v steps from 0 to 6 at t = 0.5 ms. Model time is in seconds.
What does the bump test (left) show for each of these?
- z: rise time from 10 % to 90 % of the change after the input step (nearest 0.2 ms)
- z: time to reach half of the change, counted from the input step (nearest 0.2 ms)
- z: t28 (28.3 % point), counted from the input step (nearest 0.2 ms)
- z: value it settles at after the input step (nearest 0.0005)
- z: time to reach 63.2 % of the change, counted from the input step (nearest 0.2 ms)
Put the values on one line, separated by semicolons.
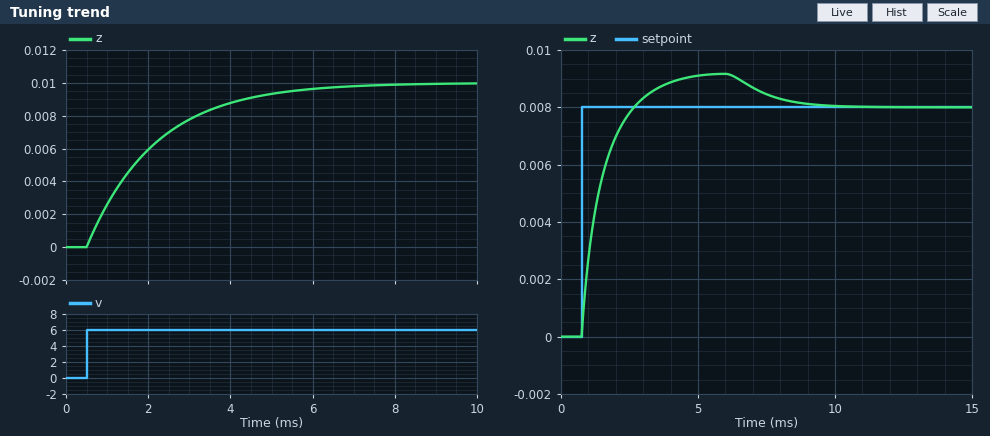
3.6 ms; 1.2 ms; 0.6 ms; 0.0100; 1.6 ms
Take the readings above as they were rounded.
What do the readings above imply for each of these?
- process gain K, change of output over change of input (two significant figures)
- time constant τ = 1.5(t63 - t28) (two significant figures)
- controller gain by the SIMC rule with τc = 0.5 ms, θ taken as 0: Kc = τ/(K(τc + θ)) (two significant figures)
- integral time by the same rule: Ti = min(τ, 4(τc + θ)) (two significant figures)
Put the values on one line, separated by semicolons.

0.0017; 1.5 ms; 1800; 1.5 ms
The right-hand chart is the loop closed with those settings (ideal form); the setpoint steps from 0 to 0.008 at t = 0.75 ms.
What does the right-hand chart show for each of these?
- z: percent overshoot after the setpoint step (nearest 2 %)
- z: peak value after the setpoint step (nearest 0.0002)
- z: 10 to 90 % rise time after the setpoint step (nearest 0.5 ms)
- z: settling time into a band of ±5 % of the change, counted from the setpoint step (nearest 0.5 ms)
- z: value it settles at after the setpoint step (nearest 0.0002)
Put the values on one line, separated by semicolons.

14 %; 0.0092; 1.5 ms; 7.0 ms; 0.0080
